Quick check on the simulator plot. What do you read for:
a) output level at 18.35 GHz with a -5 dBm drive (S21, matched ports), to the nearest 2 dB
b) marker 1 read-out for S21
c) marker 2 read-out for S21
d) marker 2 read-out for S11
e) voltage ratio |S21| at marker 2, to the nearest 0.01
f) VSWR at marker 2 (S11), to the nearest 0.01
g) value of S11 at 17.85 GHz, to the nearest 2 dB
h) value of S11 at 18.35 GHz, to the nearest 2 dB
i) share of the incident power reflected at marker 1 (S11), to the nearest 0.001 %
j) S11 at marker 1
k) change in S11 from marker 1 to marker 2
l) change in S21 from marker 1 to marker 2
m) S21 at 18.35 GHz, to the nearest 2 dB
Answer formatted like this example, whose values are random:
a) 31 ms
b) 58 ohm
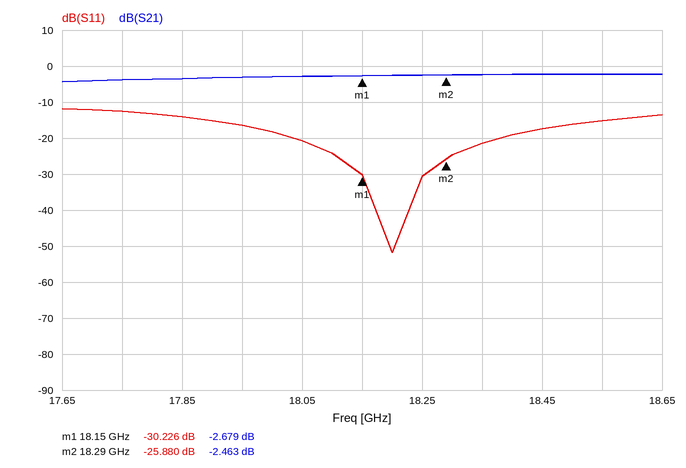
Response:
a) -8 dBm
b) -2.679 dB
c) -2.463 dB
d) -25.880 dB
e) 0.75
f) 1.11
g) -14 dB
h) -22 dB
i) 0.095 %
j) -30.226 dB
k) 4.346 dB
l) 0.216 dB
m) -2 dB
